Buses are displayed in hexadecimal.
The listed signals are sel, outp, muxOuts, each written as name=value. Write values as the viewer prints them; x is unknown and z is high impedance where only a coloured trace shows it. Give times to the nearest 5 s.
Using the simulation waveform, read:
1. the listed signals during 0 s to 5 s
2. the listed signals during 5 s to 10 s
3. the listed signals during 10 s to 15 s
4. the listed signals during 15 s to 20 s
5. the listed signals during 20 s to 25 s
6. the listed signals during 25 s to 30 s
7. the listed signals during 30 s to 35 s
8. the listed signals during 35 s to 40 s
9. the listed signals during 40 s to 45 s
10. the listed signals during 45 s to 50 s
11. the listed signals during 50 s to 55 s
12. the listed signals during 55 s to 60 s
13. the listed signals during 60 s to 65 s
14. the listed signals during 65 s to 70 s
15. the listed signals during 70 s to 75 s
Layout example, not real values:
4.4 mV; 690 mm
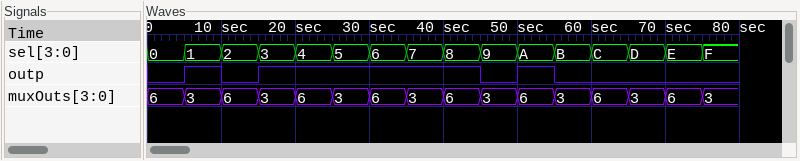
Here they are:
sel=0, outp=0, muxOuts=6; sel=1, outp=1, muxOuts=3; sel=2, outp=0, muxOuts=6; sel=3, outp=1, muxOuts=3; sel=4, outp=1, muxOuts=6; sel=5, outp=1, muxOuts=3; sel=6, outp=1, muxOuts=6; sel=7, outp=1, muxOuts=3; sel=8, outp=1, muxOuts=6; sel=9, outp=0, muxOuts=3; sel=A, outp=1, muxOuts=6; sel=B, outp=0, muxOuts=3; sel=C, outp=0, muxOuts=6; sel=D, outp=0, muxOuts=3; sel=E, outp=0, muxOuts=6
